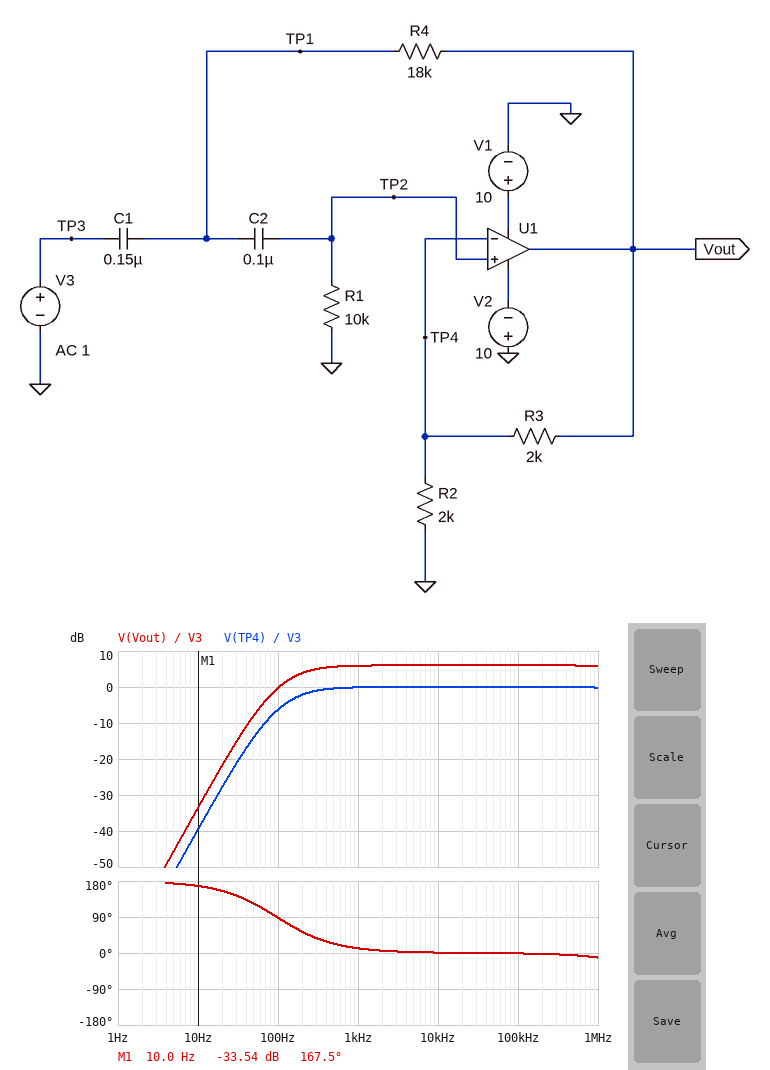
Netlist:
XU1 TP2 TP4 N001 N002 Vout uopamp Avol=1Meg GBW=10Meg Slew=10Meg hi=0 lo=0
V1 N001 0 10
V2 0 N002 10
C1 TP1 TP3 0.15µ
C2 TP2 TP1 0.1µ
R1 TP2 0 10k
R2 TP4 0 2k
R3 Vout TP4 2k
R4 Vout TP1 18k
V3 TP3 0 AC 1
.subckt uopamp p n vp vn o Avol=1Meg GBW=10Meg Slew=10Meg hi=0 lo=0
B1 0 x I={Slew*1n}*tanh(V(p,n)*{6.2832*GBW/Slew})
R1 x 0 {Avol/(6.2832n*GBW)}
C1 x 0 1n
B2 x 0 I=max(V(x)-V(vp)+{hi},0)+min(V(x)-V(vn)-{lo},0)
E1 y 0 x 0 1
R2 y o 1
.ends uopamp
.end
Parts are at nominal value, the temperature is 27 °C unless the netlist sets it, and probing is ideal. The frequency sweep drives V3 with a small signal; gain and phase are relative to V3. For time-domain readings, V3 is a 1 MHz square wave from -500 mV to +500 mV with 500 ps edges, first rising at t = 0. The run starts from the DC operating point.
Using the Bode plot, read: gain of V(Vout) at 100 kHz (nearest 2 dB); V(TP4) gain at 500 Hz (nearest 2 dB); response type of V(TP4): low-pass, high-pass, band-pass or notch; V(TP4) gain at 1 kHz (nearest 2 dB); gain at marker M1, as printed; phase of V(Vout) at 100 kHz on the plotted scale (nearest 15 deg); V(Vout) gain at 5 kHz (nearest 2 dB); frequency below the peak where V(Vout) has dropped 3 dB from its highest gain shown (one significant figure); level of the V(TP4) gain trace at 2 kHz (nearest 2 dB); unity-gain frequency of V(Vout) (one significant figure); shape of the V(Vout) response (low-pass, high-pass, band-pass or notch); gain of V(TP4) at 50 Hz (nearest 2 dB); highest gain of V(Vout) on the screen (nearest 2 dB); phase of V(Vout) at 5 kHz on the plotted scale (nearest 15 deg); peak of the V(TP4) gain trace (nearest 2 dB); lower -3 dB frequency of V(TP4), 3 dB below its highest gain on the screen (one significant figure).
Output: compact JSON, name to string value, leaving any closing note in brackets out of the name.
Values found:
{"gain of V(Vout) at 100 kHz": "6 dB", "V(TP4) gain at 500 Hz": "0 dB", "response type of V(TP4): low-pass, high-pass, band-pass or notch": "high-pass", "V(TP4) gain at 1 kHz": "0 dB", "gain at marker M1, as printed": "-33.54 dB", "phase of V(Vout) at 100 kHz on the plotted scale": "0 deg", "V(Vout) gain at 5 kHz": "6 dB", "frequency below the peak where V(Vout) has dropped 3 dB from its highest gain shown": "200 Hz", "level of the V(TP4) gain trace at 2 kHz": "0 dB", "unity-gain frequency of V(Vout)": "100 Hz", "shape of the V(Vout) response": "high-pass", "gain of V(TP4) at 50 Hz": "-14 dB", "highest gain of V(Vout) on the screen": "6 dB", "phase of V(Vout) at 5 kHz on the plotted scale": "0 deg", "peak of the V(TP4) gain trace": "0 dB", "lower -3 dB frequency of V(TP4), 3 dB below its highest gain on the screen": "200 Hz"}
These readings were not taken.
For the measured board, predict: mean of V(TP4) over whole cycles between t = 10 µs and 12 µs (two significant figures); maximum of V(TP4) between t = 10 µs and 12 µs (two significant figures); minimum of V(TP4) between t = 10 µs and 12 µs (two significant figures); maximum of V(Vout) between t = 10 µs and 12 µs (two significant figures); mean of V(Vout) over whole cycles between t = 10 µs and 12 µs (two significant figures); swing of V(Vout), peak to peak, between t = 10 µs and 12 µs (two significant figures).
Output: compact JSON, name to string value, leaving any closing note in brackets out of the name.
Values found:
{"mean of V(TP4) over whole cycles between t = 10 µs and 12 µs": "490 mV", "maximum of V(TP4) between t = 10 µs and 12 µs": "990 mV", "minimum of V(TP4) between t = 10 µs and 12 µs": "-7.7 mV", "maximum of V(Vout) between t = 10 µs and 12 µs": "2.0 V", "mean of V(Vout) over whole cycles between t = 10 µs and 12 µs": "990 mV", "swing of V(Vout), peak to peak, between t = 10 µs and 12 µs": "2.0 V"}
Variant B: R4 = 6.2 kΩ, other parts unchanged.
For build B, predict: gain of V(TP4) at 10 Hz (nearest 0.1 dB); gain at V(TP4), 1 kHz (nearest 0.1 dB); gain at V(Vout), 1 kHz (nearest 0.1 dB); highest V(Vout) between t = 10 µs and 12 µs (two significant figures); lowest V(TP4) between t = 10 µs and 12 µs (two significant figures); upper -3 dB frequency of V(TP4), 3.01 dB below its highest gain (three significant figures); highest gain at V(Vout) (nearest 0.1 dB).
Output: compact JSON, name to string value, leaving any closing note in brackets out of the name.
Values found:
{"gain of V(TP4) at 10 Hz": "-48.7 dB", "gain at V(TP4), 1 kHz": "0.2 dB", "gain at V(Vout), 1 kHz": "6.2 dB", "highest V(Vout) between t = 10 µs and 12 µs": "2.0 V", "lowest V(TP4) between t = 10 µs and 12 µs": "-3.6 mV", "upper -3 dB frequency of V(TP4), 3.01 dB below its highest gain": "306 Hz", "highest gain at V(Vout)": "11.3 dB"}
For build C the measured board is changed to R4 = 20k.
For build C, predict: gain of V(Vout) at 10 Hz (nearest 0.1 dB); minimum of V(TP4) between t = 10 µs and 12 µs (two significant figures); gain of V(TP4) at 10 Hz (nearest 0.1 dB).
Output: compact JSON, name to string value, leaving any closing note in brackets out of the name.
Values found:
{"gain of V(Vout) at 10 Hz": "-32.7 dB", "minimum of V(TP4) between t = 10 µs and 12 µs": "-7.9 mV", "gain of V(TP4) at 10 Hz": "-38.7 dB"}
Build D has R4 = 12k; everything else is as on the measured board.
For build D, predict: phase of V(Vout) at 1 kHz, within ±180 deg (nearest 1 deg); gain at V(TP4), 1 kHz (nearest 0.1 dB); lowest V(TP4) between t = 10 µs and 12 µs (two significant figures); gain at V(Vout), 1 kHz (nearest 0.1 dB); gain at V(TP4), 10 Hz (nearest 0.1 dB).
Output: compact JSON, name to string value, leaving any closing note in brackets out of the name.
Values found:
{"phase of V(Vout) at 1 kHz, within ±180 deg": "10 deg", "gain at V(TP4), 1 kHz": "0 dB", "lowest V(TP4) between t = 10 µs and 12 µs": "-6.6 mV", "gain at V(Vout), 1 kHz": "6.0 dB", "gain at V(TP4), 10 Hz": "-43.0 dB"}
